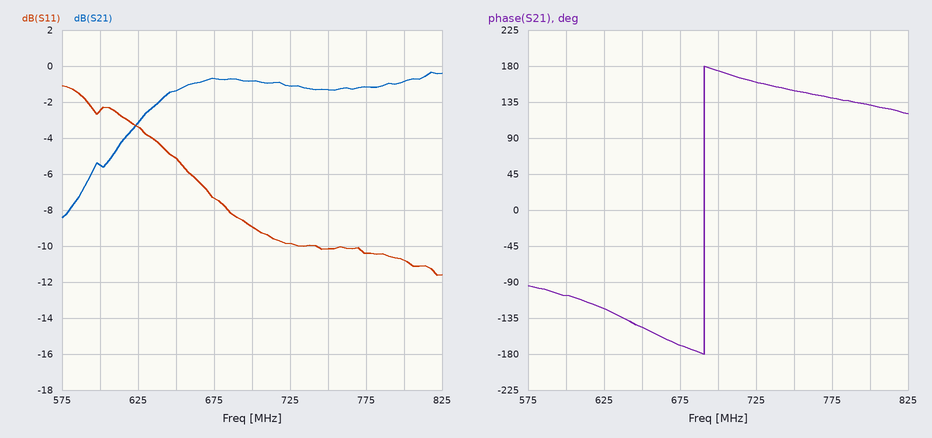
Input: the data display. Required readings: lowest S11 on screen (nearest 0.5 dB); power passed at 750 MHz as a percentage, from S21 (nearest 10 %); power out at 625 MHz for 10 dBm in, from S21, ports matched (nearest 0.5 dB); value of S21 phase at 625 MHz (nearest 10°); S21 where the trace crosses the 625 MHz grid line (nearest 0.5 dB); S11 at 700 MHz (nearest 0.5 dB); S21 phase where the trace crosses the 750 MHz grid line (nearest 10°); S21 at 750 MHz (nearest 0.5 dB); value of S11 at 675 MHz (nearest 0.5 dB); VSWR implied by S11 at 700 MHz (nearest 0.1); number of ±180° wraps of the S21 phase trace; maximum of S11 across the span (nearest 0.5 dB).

-11.5 dB
70 %
7.0 dBm
-120°
-3.0 dB
-9.0 dB
150°
-1.5 dB
-7.5 dB
2.1
1
-1.0 dB
